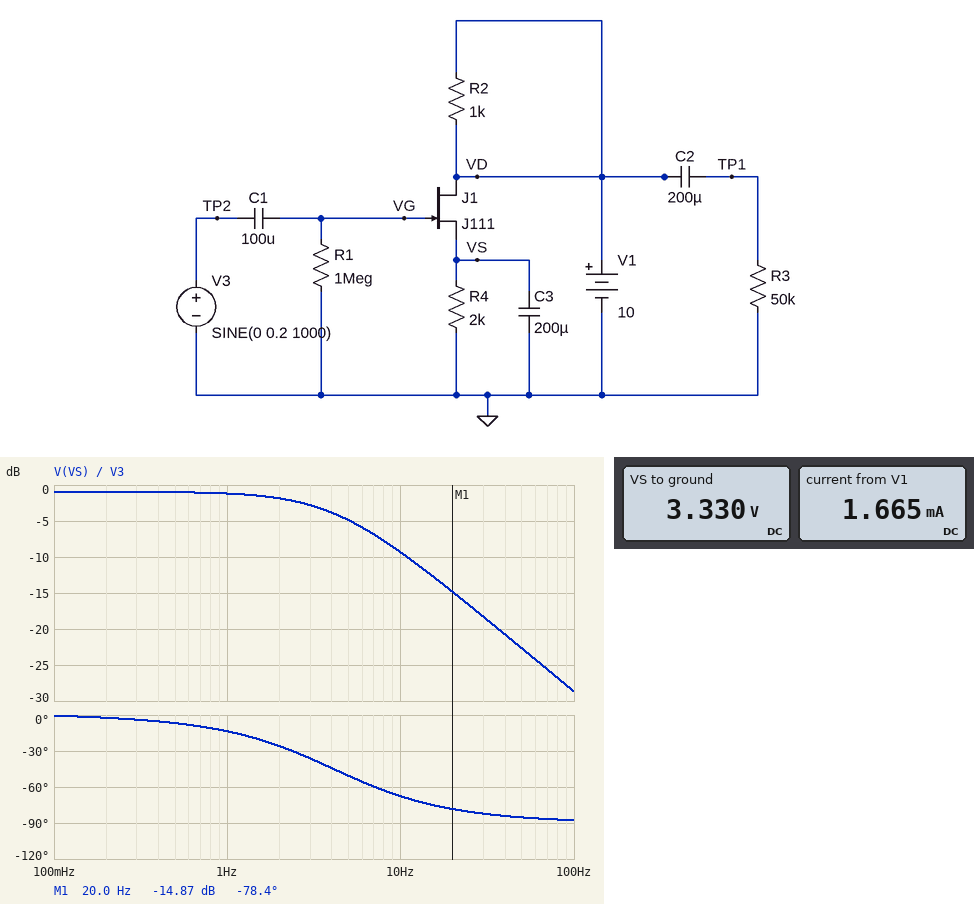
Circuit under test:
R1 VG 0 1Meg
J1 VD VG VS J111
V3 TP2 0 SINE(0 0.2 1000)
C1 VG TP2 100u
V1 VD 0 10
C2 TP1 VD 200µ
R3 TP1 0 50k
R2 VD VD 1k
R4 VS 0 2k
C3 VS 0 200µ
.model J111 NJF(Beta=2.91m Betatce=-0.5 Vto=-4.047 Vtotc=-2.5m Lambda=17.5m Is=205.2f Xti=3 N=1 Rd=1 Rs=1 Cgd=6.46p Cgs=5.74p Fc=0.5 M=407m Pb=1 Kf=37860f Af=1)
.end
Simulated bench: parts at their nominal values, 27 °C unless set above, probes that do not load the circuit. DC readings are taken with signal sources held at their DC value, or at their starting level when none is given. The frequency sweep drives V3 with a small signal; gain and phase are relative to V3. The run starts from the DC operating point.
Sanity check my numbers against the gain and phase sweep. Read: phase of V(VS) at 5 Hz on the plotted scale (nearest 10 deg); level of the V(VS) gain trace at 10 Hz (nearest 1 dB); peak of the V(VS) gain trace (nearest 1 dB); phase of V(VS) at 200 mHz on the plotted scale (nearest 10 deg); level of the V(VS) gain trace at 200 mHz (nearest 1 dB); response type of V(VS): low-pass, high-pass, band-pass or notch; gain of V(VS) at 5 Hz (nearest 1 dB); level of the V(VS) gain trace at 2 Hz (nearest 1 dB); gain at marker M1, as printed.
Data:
-50 deg
-9 dB
-1 dB
0 deg
-1 dB
low-pass
-5 dB
-2 dB
-14.87 dB
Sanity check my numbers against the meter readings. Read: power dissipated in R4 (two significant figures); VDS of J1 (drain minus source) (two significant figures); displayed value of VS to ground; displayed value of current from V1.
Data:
5.5 mW
6.7 V
3.330 V
1.665 mA
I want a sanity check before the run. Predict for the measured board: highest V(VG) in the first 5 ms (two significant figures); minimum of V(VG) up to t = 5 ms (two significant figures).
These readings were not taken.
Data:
200 mV
-200 mV
